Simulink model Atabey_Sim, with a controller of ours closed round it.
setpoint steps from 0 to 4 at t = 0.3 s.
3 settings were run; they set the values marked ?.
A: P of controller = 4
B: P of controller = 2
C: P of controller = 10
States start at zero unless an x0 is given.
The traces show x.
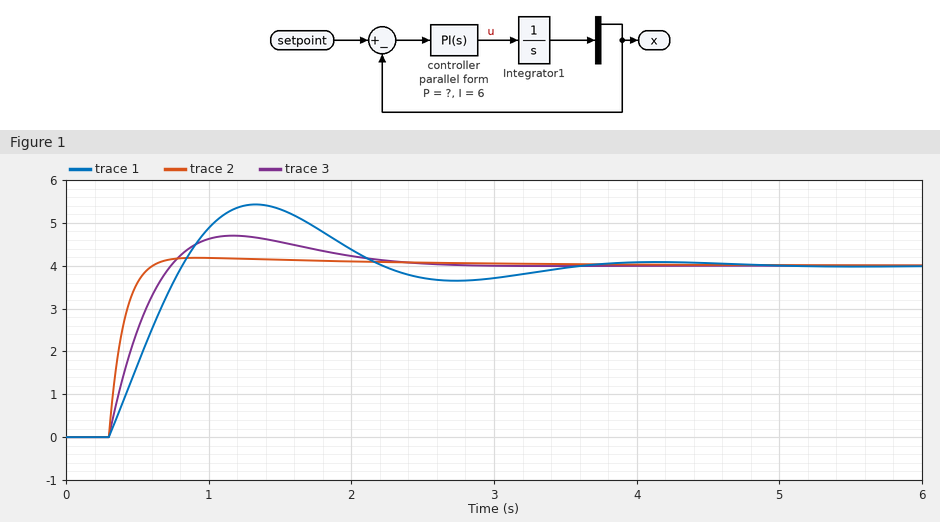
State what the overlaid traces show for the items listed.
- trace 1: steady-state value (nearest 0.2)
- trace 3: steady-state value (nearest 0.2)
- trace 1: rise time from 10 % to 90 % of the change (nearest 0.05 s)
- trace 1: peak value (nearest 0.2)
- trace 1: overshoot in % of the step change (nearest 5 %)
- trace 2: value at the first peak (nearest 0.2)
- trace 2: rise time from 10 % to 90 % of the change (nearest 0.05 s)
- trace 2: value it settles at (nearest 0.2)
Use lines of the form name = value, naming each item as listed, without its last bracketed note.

trace 1: steady-state value = 4.0
trace 3: steady-state value = 4.0
trace 1: rise time from 10 % to 90 % of the change = 0.40 s
trace 1: peak value = 5.4
trace 1: overshoot in % of the step change = 35 %
trace 2: value at the first peak = 4.2
trace 2: rise time from 10 % to 90 % of the change = 0.20 s
trace 2: value it settles at = 4.0
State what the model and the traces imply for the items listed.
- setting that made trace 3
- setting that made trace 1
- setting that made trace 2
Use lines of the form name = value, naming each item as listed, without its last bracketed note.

setting that made trace 3 = A
setting that made trace 1 = B
setting that made trace 2 = C
